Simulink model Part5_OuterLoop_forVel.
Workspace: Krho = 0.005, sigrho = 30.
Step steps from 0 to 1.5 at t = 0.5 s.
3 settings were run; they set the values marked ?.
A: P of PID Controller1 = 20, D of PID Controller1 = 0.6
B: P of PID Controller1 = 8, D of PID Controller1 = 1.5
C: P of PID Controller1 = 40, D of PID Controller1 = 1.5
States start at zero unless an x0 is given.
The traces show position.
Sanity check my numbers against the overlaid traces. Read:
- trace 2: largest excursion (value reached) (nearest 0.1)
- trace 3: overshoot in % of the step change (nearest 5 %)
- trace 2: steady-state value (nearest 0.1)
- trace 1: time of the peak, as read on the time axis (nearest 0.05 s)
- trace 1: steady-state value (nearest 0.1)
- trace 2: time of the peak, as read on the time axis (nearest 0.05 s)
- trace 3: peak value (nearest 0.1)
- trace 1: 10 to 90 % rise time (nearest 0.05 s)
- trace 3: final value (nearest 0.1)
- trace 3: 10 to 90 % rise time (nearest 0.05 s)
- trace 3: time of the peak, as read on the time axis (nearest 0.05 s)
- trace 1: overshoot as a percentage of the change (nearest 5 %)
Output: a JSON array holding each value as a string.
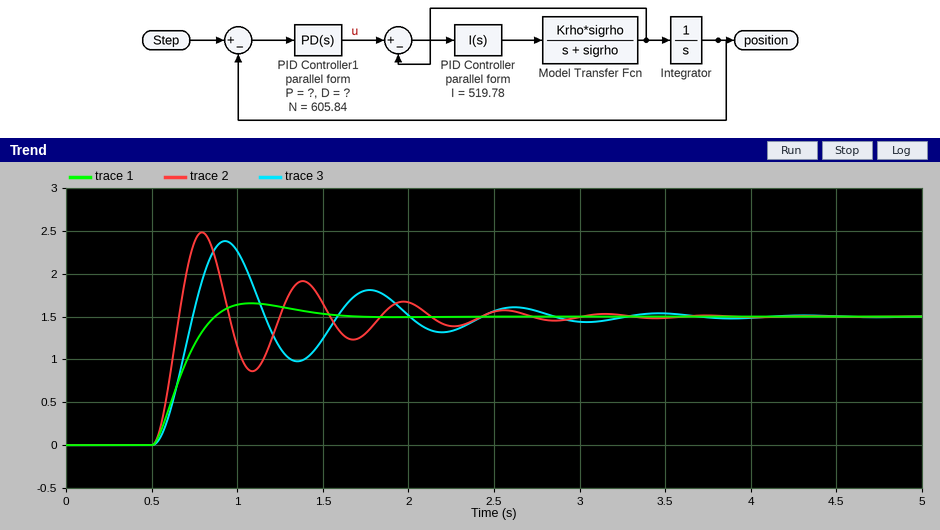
["2.5", "60 %", "1.5", "1.10 s", "1.5", "0.80 s", "2.4", "0.25 s", "1.5", "0.15 s", "0.95 s", "10 %"]
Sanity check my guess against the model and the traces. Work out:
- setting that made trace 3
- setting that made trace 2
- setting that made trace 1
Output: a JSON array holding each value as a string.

["A", "C", "B"]
